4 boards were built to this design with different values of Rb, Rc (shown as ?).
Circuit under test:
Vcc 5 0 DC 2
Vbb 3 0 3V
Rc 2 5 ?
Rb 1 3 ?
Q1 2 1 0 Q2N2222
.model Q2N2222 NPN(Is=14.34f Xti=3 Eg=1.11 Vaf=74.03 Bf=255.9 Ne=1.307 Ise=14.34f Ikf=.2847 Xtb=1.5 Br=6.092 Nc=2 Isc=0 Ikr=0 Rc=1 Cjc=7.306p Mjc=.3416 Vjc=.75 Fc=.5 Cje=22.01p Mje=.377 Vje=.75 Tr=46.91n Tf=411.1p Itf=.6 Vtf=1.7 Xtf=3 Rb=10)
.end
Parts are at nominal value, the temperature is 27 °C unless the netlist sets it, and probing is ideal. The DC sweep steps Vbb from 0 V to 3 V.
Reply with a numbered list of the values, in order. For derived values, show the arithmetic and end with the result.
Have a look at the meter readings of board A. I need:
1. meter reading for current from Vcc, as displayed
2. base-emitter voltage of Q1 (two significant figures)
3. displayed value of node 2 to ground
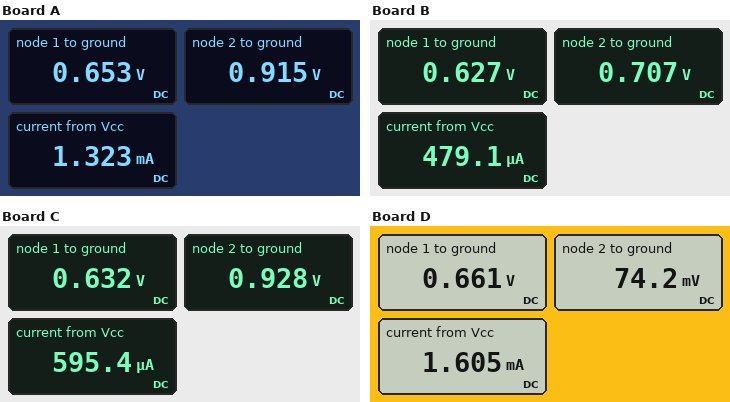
1. 1.323 mA
2. 653 mV = 650 mV
3. 0.915 V
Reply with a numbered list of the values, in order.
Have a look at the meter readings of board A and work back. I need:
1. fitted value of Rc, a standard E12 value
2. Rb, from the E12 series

1. 820 Ω
2. 270 kΩ
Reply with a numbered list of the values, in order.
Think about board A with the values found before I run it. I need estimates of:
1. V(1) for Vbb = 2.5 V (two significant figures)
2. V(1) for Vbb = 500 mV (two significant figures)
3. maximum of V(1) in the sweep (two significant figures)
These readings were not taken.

1. 650 mV
2. 490 mV
3. 650 mV
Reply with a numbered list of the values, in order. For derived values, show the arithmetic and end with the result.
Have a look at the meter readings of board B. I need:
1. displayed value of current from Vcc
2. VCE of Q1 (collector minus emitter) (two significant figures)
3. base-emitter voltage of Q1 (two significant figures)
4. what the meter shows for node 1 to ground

1. 479.1 µA
2. 707 mV = 710 mV
3. 627 mV = 630 mV
4. 0.627 V
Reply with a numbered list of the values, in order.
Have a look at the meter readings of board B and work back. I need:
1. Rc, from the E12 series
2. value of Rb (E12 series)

1. 2.7 kΩ
2. 680 kΩ
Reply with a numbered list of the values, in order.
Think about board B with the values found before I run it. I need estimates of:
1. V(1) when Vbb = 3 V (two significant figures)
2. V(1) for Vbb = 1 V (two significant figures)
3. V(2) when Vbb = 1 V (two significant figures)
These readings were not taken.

1. 630 mV
2. 580 mV
3. 1.8 V
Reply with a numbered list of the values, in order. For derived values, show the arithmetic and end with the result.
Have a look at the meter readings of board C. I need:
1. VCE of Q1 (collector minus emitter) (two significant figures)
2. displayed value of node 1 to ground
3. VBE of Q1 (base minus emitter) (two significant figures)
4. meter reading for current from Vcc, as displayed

1. 928 mV = 930 mV
2. 0.632 V
3. 632 mV = 630 mV
4. 595.4 µA
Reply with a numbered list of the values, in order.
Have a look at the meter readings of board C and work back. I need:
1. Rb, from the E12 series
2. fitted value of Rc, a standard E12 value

1. 560 kΩ
2. 1.8 kΩ
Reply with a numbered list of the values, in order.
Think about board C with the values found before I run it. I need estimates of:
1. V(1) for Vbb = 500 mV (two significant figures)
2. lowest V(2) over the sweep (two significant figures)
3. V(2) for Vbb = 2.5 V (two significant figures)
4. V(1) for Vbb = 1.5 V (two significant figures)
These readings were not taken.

1. 480 mV
2. 930 mV
3. 1.2 V
4. 600 mV
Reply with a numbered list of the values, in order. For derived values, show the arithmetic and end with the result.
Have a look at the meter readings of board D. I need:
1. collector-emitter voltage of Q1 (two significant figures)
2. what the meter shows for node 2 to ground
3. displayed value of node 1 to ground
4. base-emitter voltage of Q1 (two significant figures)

1. 74.2 mV = 74 mV
2. 74.2 mV
3. 0.661 V
4. 661 mV = 660 mV
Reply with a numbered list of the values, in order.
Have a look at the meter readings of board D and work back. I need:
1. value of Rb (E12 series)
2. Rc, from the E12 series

1. 82 kΩ
2. 1.2 kΩ
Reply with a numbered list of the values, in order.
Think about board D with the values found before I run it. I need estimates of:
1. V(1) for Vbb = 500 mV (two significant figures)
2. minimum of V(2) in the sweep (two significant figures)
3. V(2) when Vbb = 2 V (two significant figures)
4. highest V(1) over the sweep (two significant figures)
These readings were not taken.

1. 500 mV
2. 74 mV
3. 100 mV
4. 660 mV
